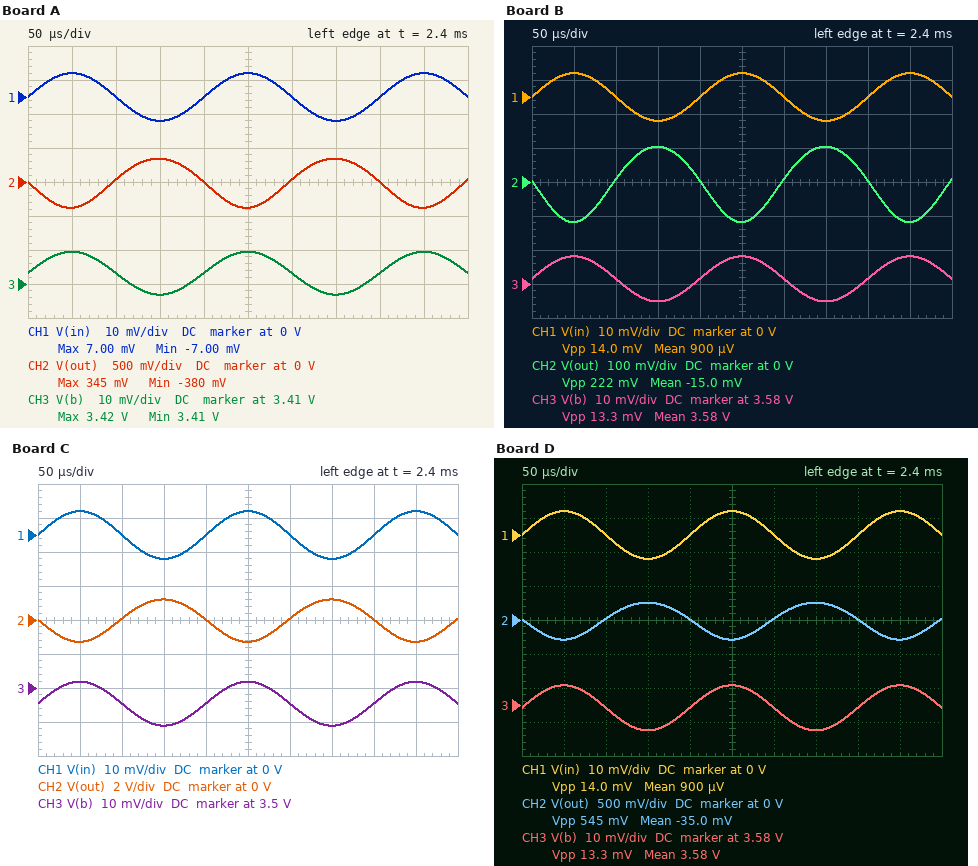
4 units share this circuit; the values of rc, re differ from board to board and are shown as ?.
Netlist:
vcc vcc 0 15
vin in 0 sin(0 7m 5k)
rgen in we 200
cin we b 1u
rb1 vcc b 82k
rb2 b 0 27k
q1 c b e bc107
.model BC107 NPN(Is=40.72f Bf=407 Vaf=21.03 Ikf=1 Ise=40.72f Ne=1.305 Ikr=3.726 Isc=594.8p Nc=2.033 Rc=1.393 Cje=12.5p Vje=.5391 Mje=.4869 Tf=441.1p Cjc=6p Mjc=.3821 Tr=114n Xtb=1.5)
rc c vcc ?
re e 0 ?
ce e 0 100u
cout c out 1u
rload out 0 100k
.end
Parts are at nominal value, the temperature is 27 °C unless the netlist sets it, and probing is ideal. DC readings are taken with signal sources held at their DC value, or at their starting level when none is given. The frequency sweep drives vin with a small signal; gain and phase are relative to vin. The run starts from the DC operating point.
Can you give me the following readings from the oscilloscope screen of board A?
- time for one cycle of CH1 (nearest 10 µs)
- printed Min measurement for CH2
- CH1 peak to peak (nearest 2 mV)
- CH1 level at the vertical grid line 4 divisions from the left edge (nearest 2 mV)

200 µs
-380 mV
14 mV
0 V
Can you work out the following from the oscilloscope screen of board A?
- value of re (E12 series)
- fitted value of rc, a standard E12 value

680 Ω
390 Ω
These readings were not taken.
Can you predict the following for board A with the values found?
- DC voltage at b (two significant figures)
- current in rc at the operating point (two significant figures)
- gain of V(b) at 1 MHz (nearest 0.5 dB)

3.4 V
4.1 mA
-1.0 dB
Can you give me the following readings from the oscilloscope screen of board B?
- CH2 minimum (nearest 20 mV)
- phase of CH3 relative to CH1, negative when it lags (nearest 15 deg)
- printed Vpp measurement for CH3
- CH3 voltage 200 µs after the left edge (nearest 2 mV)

-120 mV
0 deg
13.3 mV
3.582 V
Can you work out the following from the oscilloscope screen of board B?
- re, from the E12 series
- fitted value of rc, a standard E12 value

1.8 kΩ
270 Ω
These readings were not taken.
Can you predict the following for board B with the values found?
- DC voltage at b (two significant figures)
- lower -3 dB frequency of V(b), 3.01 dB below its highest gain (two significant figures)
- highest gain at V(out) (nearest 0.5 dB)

3.6 V
14 Hz
24.0 dB
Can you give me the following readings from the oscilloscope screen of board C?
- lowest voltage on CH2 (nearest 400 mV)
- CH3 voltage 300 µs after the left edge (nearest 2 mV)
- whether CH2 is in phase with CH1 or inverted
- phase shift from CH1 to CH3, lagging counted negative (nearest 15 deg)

-1.2 V
3.496 V
inverted
0 deg
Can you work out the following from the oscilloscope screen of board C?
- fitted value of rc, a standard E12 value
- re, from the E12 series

2.7 kΩ
1.2 kΩ
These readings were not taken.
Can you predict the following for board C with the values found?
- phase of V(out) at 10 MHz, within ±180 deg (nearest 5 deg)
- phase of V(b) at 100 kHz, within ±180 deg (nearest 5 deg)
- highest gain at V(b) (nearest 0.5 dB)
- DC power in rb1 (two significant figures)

95 deg
-5 deg
-0.5 dB
1.6 mW
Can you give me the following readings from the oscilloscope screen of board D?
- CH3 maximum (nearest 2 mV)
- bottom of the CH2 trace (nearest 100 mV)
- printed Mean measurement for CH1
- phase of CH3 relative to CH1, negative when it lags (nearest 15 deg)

3.586 V
-300 mV
900 µV
0 deg
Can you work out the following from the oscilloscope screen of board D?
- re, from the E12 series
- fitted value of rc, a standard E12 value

1.8 kΩ
680 Ω
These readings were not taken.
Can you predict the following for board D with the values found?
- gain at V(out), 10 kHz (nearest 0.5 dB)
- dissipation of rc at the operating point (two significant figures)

32.0 dB
1.8 mW
